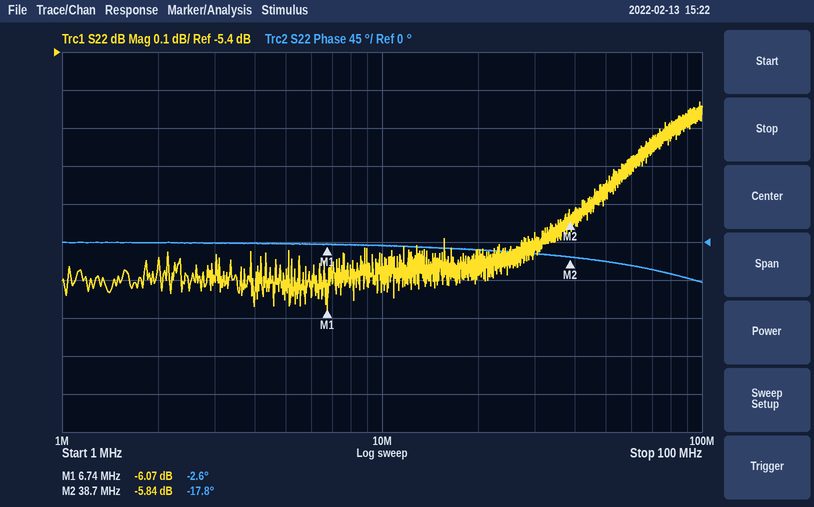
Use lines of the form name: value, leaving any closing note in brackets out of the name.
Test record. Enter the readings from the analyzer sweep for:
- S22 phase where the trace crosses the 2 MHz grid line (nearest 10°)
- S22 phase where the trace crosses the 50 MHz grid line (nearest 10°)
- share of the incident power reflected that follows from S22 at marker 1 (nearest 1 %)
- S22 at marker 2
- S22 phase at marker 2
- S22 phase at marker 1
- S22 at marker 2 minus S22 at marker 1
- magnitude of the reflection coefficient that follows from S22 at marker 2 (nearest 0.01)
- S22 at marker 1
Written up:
S22 phase where the trace crosses the 2 MHz grid line: 0°
S22 phase where the trace crosses the 50 MHz grid line: -20°
share of the incident power reflected that follows from S22 at marker 1: 25 %
S22 at marker 2: -5.84 dB
S22 phase at marker 2: -17.8°
S22 phase at marker 1: -2.6°
S22 at marker 2 minus S22 at marker 1: 0.23 dB
magnitude of the reflection coefficient that follows from S22 at marker 2: 0.51
S22 at marker 1: -6.07 dB
